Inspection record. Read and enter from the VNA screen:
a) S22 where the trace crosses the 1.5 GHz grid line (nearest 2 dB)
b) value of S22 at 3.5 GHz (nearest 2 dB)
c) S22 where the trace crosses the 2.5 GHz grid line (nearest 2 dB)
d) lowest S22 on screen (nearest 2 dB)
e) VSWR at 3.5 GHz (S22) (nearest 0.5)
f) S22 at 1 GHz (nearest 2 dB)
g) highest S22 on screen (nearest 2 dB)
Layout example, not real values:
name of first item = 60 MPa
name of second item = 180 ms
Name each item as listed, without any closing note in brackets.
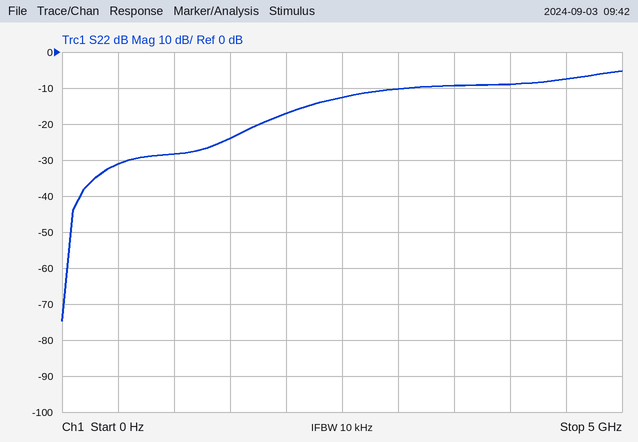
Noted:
S22 where the trace crosses the 1.5 GHz grid line = -24 dB
value of S22 at 3.5 GHz = -10 dB
S22 where the trace crosses the 2.5 GHz grid line = -12 dB
lowest S22 on screen = -74 dB
VSWR at 3.5 GHz (S22) = 2.0
S22 at 1 GHz = -28 dB
highest S22 on screen = -6 dB
